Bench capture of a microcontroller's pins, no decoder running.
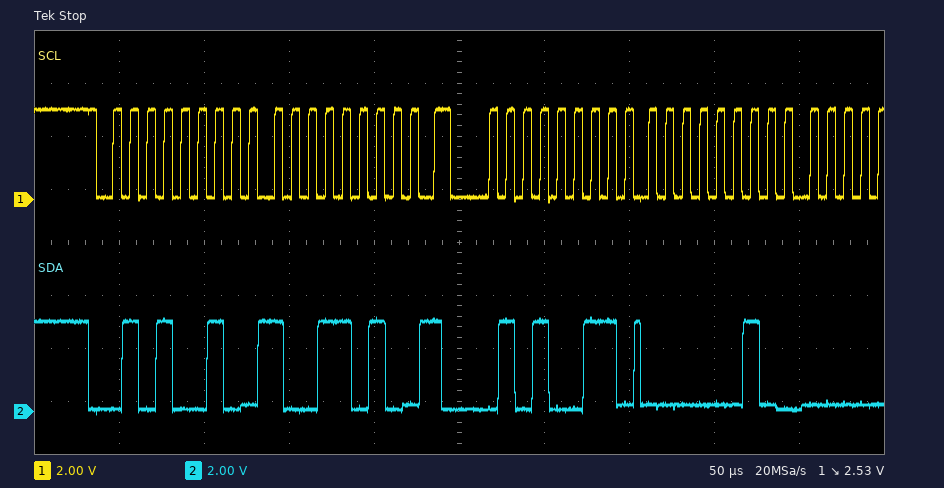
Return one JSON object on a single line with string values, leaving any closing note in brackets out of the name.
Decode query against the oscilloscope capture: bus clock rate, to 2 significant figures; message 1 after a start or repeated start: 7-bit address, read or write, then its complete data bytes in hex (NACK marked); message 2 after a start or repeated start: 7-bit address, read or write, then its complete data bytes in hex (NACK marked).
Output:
{"bus clock rate, to 2 significant figures": "100 kHz", "message 1 after a start or repeated start: 7-bit address, read or write, then its complete data bytes in hex": "0x29 write: 9A", "message 2 after a start or repeated start: 7-bit address, read or write, then its complete data bytes in hex": "0x29 read: 02"}
